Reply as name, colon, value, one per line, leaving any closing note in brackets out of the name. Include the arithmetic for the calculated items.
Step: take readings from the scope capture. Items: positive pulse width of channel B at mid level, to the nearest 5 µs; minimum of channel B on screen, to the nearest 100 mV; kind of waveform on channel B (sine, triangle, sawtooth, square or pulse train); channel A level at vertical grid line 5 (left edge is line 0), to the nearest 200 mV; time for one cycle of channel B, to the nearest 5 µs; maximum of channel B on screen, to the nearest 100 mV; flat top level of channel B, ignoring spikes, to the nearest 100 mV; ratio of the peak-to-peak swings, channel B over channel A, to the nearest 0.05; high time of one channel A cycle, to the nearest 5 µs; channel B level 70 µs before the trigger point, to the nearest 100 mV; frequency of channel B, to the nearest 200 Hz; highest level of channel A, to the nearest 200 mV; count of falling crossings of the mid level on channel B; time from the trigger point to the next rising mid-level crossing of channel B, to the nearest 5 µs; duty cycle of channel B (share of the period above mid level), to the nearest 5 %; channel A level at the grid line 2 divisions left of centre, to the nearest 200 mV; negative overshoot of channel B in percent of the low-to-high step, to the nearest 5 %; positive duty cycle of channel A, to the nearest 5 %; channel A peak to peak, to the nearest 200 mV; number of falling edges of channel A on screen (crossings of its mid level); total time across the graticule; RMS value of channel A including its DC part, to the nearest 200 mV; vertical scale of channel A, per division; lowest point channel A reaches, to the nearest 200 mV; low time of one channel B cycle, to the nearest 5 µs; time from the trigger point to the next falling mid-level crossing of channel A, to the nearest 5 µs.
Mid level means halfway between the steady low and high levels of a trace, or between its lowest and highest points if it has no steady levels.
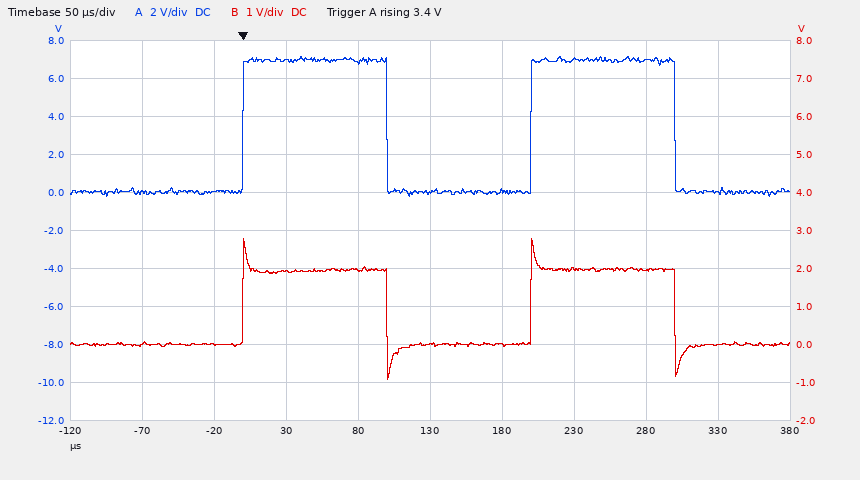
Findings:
positive pulse width of channel B at mid level, to the nearest 5 µs: 100 µs
minimum of channel B on screen, to the nearest 100 mV: -900 mV
kind of waveform on channel B: square
channel A level at vertical grid line 5 (left edge is line 0), to the nearest 200 mV: 0.0 V
time for one cycle of channel B, to the nearest 5 µs: 200 µs
maximum of channel B on screen, to the nearest 100 mV: 2.8 V
flat top level of channel B, ignoring spikes, to the nearest 100 mV: 2.0 V
ratio of the peak-to-peak swings, channel B over channel A, to the nearest 0.05: 3.7 V / 7.4 V ≈ 0.50
high time of one channel A cycle, to the nearest 5 µs: 100 µs
channel B level 70 µs before the trigger point, to the nearest 100 mV: 0.0 V
frequency of channel B, to the nearest 200 Hz: 1 / 200 µs ≈ 5.0 kHz
highest level of channel A, to the nearest 200 mV: 7.2 V
count of falling crossings of the mid level on channel B: 2
time from the trigger point to the next rising mid-level crossing of channel B, to the nearest 5 µs: 200 µs
duty cycle of channel B (share of the period above mid level), to the nearest 5 %: 100 µs / 200 µs ≈ 50 %
channel A level at the grid line 2 divisions left of centre, to the nearest 200 mV: 7.0 V
negative overshoot of channel B in percent of the low-to-high step, to the nearest 5 %: 45 %
positive duty cycle of channel A, to the nearest 5 %: 100 µs / 200 µs ≈ 50 %
channel A peak to peak, to the nearest 200 mV: 7.2 V − (-200 mV) = 7.4 V
number of falling edges of channel A on screen: 2
total time across the graticule: 500 µs
RMS value of channel A including its DC part, to the nearest 200 mV: √(0.5 × (7.2 V)² + 0.5 × (-200 mV)²) ≈ 5.09 V, so 5.0 V to the nearest 200 mV
vertical scale of channel A, per division: 2 V
lowest point channel A reaches, to the nearest 200 mV: -200 mV
low time of one channel B cycle, to the nearest 5 µs: 100 µs
time from the trigger point to the next falling mid-level crossing of channel A, to the nearest 5 µs: 100 µs
